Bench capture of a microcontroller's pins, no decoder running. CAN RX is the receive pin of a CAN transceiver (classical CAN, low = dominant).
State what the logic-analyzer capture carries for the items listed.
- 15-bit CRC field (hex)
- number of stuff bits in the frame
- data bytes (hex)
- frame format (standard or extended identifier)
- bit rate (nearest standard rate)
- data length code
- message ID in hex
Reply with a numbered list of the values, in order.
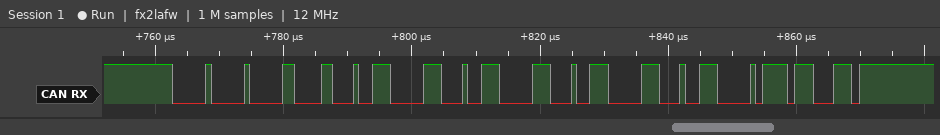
1. 0x1EE3
2. 7
3. 62 70 62 70 62 70 62 70
4. standard
5. 1000 kbit/s
6. 8
7. 0x000
